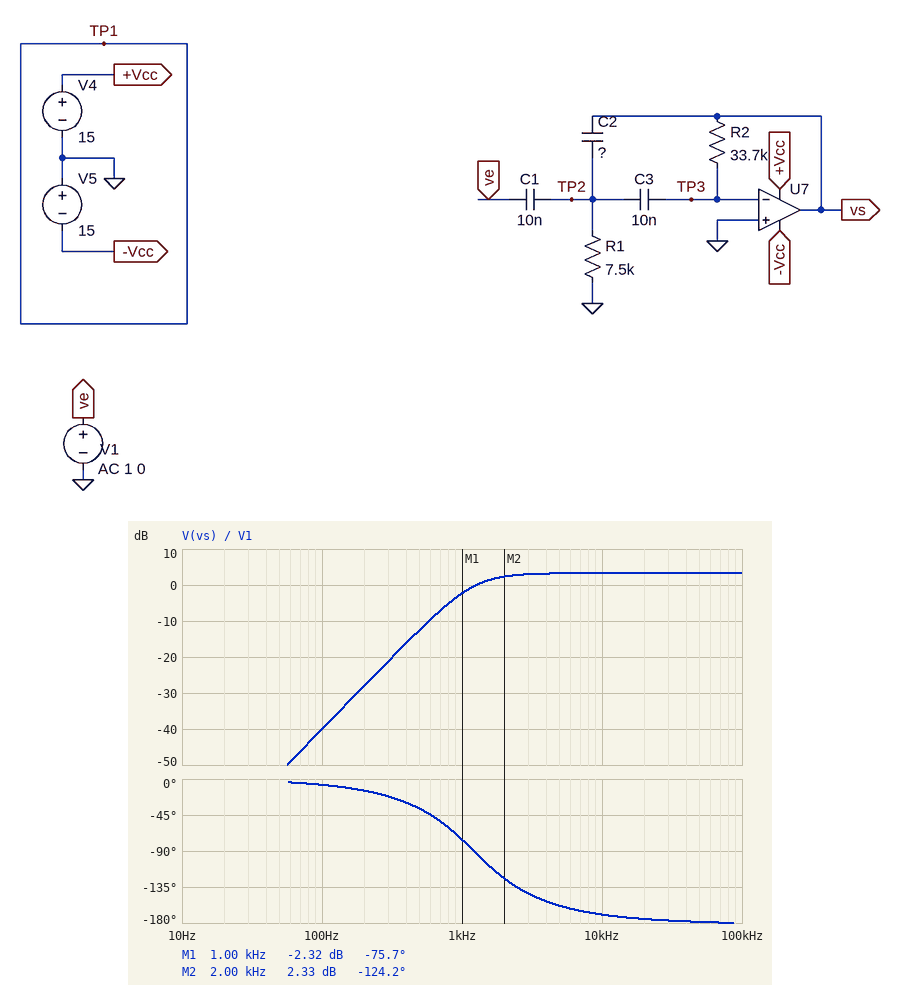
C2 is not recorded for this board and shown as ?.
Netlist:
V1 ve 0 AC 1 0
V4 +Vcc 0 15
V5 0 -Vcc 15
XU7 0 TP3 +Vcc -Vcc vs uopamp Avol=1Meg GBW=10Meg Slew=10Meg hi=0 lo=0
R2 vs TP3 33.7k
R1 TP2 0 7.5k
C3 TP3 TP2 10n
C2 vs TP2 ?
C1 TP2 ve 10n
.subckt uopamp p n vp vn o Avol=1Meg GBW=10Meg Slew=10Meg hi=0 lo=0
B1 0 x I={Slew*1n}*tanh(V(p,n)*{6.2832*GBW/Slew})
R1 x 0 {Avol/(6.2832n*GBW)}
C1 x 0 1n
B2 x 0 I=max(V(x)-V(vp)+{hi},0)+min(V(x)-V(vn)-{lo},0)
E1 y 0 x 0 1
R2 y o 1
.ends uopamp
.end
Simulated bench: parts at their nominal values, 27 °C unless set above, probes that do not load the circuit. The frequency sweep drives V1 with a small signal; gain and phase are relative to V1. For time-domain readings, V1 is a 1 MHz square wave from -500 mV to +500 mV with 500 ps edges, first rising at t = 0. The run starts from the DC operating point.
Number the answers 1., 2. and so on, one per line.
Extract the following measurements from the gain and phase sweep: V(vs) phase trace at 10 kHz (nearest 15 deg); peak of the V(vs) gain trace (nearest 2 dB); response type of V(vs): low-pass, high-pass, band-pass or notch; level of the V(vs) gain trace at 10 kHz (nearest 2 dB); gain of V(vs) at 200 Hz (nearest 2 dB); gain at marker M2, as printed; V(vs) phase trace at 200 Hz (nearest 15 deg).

1. -165 deg
2. 4 dB
3. high-pass
4. 4 dB
5. -28 dB
6. 2.33 dB
7. -15 deg
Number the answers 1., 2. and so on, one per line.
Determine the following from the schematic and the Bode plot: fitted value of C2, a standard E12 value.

1. 6.8 nF
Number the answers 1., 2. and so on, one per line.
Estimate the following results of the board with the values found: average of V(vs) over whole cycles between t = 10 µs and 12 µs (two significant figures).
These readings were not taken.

1. -640 mV
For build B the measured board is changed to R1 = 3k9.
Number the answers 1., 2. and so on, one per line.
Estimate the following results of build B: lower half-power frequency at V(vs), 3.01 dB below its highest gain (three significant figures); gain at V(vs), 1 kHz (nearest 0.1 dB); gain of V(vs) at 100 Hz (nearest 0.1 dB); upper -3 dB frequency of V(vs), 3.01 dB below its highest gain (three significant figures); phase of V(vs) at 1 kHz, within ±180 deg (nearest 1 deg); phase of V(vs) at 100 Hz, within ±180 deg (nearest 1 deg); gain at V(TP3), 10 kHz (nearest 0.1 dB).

1. 1.47 kHz
2. -5.0 dB
3. -45.7 dB
4. 4.52 MHz
5. -45 deg
6. -4 deg
7. -56.6 dB
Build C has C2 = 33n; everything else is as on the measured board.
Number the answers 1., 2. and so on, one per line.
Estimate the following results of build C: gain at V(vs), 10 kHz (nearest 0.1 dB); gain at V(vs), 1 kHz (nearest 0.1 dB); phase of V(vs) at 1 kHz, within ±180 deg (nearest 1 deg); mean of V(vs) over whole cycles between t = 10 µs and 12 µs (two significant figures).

1. -10.4 dB
2. -10.6 dB
3. -133 deg
4. -140 mV
